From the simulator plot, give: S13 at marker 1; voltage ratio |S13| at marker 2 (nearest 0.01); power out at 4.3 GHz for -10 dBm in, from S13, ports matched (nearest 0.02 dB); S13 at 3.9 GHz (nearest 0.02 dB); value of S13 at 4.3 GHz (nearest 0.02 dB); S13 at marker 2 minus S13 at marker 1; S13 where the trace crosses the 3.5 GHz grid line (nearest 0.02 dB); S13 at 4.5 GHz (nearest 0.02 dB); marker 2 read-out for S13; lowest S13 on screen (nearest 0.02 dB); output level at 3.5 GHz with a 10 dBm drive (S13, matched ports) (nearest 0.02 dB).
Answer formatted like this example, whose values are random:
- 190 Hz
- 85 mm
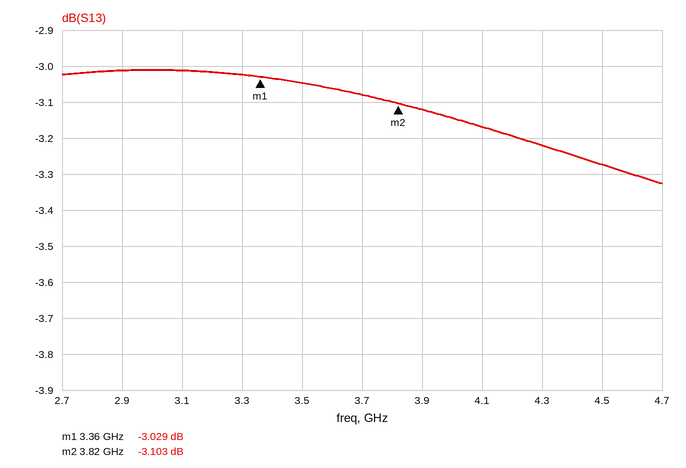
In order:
- -3.029 dB
- 0.70
- -13.22 dBm
- -3.12 dB
- -3.22 dB
- -0.074 dB
- -3.04 dB
- -3.28 dB
- -3.103 dB
- -3.32 dB
- 6.96 dBm
